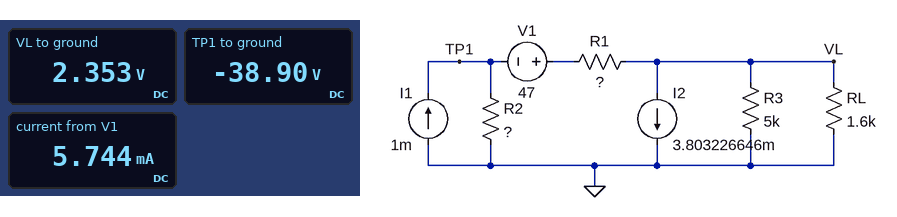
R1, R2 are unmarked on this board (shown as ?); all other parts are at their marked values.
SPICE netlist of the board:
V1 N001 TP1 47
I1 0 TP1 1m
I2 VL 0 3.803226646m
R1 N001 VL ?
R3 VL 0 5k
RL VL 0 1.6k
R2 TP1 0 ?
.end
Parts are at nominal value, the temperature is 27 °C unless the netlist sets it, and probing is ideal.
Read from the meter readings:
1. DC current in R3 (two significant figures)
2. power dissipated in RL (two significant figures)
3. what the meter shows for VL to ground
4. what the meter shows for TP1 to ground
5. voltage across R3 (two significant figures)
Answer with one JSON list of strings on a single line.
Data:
["470 µA", "3.5 mW", "2.353 V", "-38.90 V", "2.4 V"]
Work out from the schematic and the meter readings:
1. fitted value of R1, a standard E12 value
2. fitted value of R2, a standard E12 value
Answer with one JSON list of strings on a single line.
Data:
["1 kΩ", "8.2 kΩ"]
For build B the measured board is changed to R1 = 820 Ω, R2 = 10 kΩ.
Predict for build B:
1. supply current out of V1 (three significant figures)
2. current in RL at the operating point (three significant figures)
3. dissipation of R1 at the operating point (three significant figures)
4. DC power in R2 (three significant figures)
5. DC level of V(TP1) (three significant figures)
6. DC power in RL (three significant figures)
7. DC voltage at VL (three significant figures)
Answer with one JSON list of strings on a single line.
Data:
["5.12 mA", "998 µA", "21.5 mW", "170 mW", "-41.2 V", "1.59 mW", "1.60 V"]
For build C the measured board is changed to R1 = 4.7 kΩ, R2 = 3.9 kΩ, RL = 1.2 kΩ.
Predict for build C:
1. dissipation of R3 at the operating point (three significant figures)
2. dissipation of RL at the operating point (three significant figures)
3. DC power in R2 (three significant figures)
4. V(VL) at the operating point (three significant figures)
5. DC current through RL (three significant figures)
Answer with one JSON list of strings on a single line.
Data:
["677 µW", "2.82 mW", "86.3 mW", "1.84 V", "1.53 mA"]
